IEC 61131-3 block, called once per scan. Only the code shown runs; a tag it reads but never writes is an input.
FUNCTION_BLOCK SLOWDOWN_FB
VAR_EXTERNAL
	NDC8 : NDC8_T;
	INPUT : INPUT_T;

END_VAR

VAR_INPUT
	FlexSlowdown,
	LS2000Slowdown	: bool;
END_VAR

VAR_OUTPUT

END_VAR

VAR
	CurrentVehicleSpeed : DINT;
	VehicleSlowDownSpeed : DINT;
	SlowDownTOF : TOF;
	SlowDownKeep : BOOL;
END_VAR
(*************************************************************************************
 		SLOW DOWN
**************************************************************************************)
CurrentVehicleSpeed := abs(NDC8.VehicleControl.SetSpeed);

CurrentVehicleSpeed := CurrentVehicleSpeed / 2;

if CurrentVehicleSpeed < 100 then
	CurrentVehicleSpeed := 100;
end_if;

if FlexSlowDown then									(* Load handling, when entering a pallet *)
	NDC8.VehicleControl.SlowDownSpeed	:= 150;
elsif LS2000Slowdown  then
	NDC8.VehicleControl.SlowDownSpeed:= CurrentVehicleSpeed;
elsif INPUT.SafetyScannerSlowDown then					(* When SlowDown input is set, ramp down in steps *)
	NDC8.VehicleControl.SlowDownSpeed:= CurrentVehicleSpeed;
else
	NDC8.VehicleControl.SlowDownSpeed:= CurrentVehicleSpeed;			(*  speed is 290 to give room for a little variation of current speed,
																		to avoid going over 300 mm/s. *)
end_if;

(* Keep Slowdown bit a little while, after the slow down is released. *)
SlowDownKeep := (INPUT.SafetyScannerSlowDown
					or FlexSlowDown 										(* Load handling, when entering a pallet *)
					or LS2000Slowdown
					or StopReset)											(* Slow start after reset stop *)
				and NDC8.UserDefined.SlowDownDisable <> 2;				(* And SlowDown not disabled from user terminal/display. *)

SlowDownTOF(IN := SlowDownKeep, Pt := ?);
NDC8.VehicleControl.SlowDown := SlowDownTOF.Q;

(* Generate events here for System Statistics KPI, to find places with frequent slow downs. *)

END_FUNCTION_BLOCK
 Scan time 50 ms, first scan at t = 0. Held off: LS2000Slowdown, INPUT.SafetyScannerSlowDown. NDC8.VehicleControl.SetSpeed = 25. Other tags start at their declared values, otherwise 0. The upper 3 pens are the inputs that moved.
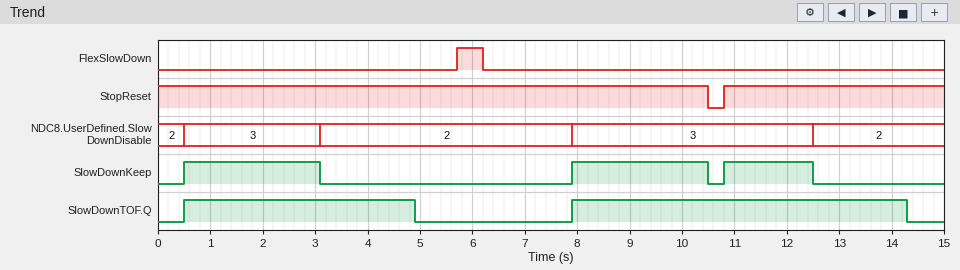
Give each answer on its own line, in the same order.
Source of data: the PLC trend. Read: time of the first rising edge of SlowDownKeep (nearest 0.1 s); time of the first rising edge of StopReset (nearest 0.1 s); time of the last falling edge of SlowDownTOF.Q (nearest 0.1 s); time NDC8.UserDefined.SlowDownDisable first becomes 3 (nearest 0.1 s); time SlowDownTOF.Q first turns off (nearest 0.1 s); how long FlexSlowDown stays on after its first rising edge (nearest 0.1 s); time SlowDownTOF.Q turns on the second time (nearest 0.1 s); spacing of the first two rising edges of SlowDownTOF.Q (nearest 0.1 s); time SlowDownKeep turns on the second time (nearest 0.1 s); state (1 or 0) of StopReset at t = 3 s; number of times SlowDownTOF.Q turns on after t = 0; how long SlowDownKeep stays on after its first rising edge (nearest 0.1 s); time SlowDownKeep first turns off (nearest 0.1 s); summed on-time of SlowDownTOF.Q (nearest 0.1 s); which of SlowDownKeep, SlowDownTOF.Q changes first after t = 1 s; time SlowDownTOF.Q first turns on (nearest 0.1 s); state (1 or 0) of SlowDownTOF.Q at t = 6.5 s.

0.5 s
10.8 s
14.3 s
0.5 s
4.9 s
0.5 s
7.9 s
7.4 s
7.9 s
1
2
2.6 s
3.1 s
10.8 s
SlowDownKeep
0.5 s
0
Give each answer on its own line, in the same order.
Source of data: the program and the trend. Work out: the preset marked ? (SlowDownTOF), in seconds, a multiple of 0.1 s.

1.8 s
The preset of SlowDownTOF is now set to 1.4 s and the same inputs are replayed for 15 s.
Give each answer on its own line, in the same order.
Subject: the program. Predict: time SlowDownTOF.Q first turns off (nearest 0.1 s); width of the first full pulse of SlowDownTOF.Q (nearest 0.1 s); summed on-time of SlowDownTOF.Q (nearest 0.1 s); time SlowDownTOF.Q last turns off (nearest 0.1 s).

4.5 s
4.0 s
10.0 s
13.9 s
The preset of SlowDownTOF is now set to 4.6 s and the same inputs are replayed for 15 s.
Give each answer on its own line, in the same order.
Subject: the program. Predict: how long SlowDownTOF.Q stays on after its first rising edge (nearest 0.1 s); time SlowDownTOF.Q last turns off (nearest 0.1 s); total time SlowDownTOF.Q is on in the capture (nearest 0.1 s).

7.2 s
7.7 s
14.3 s
